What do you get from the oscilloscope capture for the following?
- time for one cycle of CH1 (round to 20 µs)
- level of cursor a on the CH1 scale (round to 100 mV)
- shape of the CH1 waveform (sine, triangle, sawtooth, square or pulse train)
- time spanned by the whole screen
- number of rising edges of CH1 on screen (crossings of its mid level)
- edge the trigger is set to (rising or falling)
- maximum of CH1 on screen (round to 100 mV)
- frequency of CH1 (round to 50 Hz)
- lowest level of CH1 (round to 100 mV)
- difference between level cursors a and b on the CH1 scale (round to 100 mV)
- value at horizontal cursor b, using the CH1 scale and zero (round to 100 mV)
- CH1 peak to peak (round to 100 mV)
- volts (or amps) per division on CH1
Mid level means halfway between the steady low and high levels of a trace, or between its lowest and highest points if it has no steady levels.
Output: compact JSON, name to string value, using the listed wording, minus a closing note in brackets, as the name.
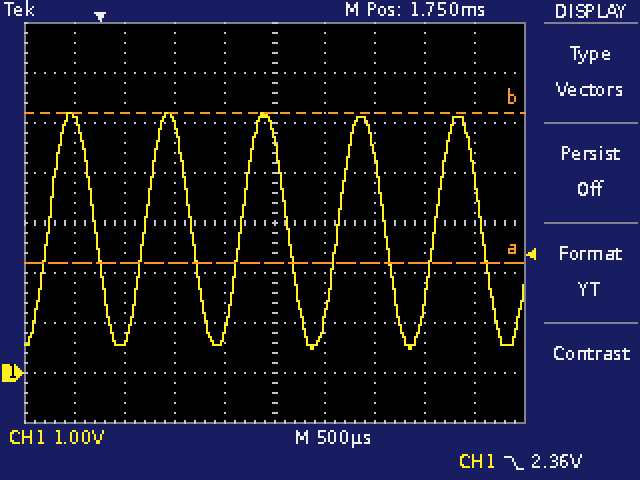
{"time for one cycle of CH1": "960 µs", "level of cursor a on the CH1 scale": "2.2 V", "shape of the CH1 waveform": "sine", "time spanned by the whole screen": "5 ms", "number of rising edges of CH1 on screen": "5", "edge the trigger is set to": "falling", "maximum of CH1 on screen": "5.2 V", "frequency of CH1": "1.05 kHz", "lowest level of CH1": "500 mV", "difference between level cursors a and b on the CH1 scale": "3.0 V", "value at horizontal cursor b, using the CH1 scale and zero": "5.2 V", "CH1 peak to peak": "4.7 V", "volts (or amps) per division on CH1": "1 V"}
